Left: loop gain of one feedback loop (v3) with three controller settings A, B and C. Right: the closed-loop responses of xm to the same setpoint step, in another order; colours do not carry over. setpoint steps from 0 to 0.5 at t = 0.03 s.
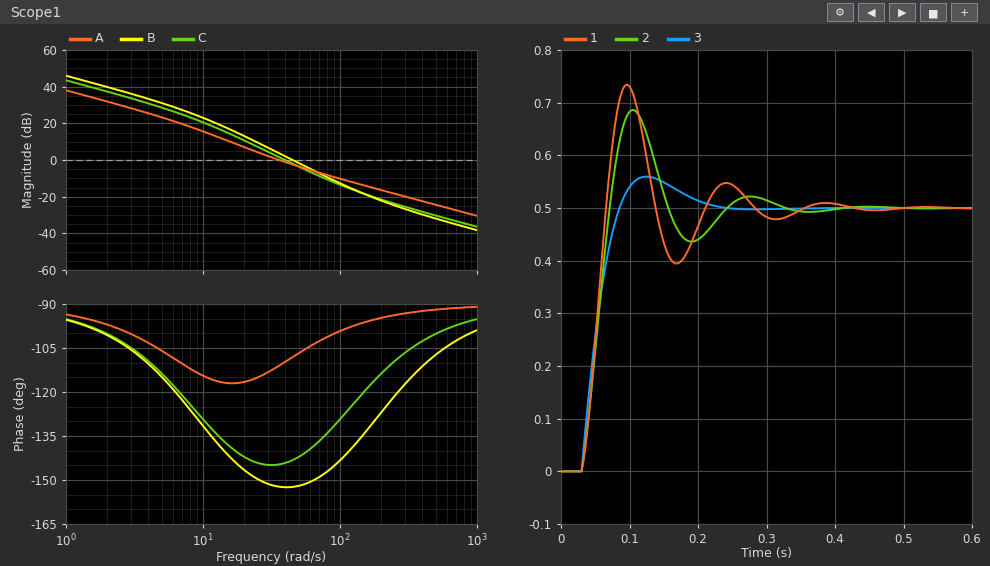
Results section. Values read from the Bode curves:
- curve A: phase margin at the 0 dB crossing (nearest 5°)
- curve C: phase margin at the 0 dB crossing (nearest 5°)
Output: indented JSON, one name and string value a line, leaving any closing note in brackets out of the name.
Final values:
{
  "curve A: phase margin at the 0 dB crossing": "70°",
  "curve C: phase margin at the 0 dB crossing": "35°"
}
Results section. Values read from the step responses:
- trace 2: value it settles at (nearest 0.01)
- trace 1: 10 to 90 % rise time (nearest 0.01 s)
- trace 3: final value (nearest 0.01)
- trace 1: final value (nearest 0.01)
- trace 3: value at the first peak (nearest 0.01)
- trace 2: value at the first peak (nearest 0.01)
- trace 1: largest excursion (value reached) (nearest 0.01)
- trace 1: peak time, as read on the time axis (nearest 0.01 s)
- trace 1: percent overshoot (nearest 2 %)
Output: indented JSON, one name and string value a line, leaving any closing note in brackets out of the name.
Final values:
{
  "trace 2: value it settles at": "0.50",
  "trace 1: 10 to 90 % rise time": "0.03 s",
  "trace 3: final value": "0.50",
  "trace 1: final value": "0.50",
  "trace 3: value at the first peak": "0.56",
  "trace 2: value at the first peak": "0.69",
  "trace 1: largest excursion (value reached)": "0.73",
  "trace 1: peak time, as read on the time axis": "0.10 s",
  "trace 1: percent overshoot": "46 %"
}
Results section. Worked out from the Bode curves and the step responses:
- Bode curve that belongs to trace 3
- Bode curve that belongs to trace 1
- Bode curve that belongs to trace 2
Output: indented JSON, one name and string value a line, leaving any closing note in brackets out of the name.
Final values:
{
  "Bode curve that belongs to trace 3": "A",
  "Bode curve that belongs to trace 1": "B",
  "Bode curve that belongs to trace 2": "C"
}
